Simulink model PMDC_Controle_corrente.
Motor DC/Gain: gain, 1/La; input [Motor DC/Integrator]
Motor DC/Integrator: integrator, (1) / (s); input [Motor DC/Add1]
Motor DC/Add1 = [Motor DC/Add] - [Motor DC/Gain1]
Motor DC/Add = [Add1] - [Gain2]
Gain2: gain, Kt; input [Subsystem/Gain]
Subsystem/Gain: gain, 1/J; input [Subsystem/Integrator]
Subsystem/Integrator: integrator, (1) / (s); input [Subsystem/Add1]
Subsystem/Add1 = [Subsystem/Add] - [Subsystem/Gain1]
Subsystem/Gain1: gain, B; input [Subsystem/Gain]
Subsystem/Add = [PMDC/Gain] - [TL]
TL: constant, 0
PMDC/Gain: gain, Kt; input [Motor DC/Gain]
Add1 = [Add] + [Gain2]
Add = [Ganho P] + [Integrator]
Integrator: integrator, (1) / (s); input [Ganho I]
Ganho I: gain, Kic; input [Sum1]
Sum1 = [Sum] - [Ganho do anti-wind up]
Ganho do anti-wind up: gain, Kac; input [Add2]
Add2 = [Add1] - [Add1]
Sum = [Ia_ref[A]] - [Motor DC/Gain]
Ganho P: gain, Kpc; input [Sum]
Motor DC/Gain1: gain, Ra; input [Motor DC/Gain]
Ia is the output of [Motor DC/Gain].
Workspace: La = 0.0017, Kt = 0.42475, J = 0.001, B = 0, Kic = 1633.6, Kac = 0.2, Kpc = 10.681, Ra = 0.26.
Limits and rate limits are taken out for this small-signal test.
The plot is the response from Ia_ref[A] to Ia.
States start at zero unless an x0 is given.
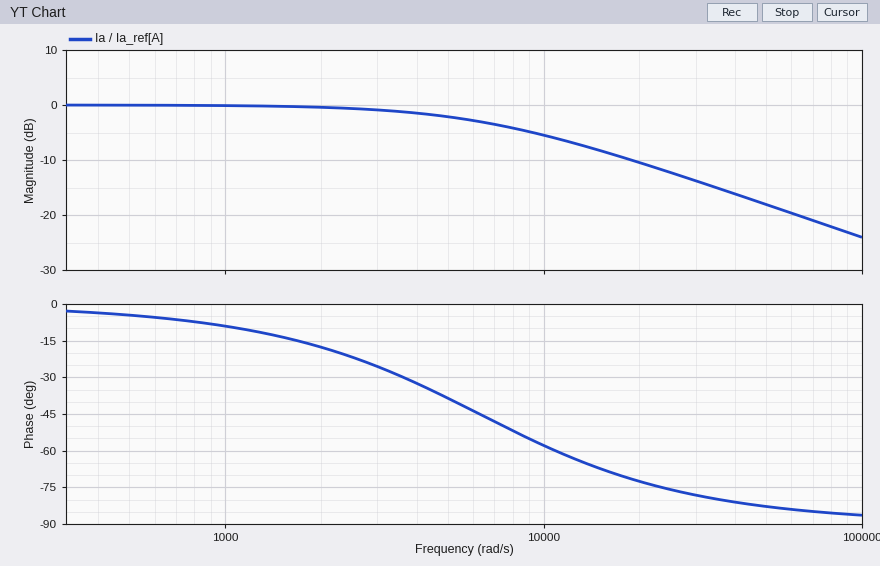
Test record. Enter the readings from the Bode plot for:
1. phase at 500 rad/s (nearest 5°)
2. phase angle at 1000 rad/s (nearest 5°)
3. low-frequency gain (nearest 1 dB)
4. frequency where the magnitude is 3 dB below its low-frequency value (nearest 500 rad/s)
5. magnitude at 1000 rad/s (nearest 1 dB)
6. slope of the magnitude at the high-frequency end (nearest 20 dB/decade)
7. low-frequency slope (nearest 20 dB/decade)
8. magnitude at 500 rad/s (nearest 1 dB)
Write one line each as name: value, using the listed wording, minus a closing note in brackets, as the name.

phase at 500 rad/s: -5°
phase angle at 1000 rad/s: -10°
low-frequency gain: 0 dB
frequency where the magnitude is 3 dB below its low-frequency value: 6500 rad/s
magnitude at 1000 rad/s: 0 dB
slope of the magnitude at the high-frequency end: -20 dB/decade
low-frequency slope: 0 dB/decade
magnitude at 500 rad/s: 0 dB
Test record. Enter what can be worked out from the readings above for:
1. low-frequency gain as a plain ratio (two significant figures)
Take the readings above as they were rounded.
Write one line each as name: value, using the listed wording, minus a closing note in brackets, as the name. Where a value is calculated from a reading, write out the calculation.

low-frequency gain as a plain ratio: 10^(0 / 20) = 1.0
